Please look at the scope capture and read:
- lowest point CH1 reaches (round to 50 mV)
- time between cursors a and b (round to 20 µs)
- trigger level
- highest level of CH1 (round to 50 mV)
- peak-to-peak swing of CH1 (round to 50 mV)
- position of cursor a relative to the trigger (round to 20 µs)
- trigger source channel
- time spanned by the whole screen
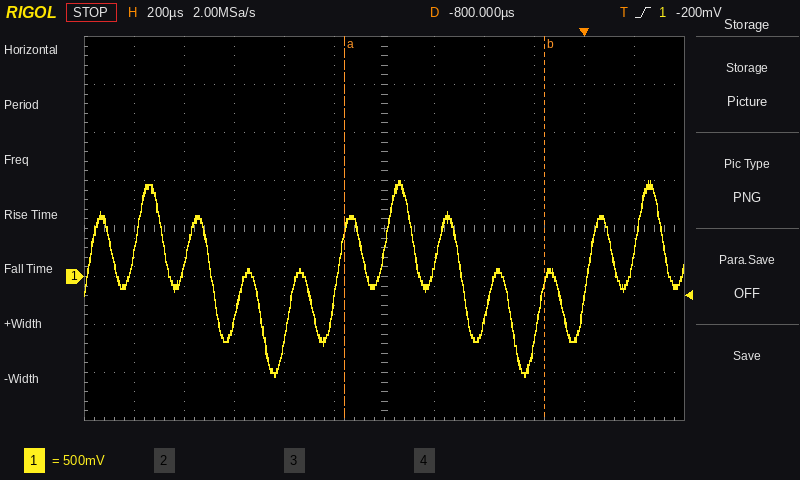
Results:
-1.05 V
800 µs
-200 mV
1.00 V
2.05 V
-960 µs
CH1
2.4 ms
